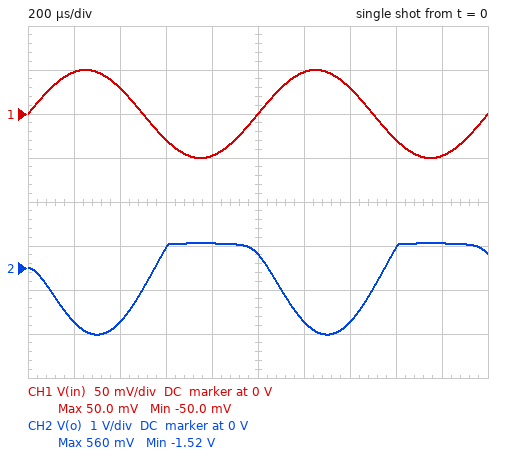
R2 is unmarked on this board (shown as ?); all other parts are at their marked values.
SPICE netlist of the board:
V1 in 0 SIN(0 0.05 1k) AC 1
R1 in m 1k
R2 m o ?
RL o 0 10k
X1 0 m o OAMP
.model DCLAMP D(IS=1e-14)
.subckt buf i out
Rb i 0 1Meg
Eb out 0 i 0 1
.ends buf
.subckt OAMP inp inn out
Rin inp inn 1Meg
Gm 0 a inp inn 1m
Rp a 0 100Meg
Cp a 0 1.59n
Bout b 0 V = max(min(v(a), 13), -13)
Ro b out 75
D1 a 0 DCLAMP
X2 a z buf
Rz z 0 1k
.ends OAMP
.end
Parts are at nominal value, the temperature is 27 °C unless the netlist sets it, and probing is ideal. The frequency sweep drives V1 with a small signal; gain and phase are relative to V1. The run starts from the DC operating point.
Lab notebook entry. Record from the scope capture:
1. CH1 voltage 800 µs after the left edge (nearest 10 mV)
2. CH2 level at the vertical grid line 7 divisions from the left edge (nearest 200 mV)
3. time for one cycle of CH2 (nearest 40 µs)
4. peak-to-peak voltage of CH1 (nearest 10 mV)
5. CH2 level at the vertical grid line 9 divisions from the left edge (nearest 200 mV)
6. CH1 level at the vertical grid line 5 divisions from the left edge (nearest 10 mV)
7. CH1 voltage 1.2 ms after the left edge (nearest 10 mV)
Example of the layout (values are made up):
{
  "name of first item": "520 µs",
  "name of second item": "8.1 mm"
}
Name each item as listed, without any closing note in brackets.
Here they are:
{
  "CH1 voltage 800 µs after the left edge": "-50 mV",
  "CH2 level at the vertical grid line 7 divisions from the left edge": "-1.2 V",
  "time for one cycle of CH2": "1.00 ms",
  "peak-to-peak voltage of CH1": "100 mV",
  "CH2 level at the vertical grid line 9 divisions from the left edge": "600 mV",
  "CH1 level at the vertical grid line 5 divisions from the left edge": "0 V",
  "CH1 voltage 1.2 ms after the left edge": "50 mV"
}
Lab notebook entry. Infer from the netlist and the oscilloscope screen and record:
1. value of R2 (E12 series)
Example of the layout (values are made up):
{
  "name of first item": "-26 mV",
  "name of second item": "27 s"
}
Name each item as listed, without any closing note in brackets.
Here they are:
{
  "value of R2": "33 kΩ"
}
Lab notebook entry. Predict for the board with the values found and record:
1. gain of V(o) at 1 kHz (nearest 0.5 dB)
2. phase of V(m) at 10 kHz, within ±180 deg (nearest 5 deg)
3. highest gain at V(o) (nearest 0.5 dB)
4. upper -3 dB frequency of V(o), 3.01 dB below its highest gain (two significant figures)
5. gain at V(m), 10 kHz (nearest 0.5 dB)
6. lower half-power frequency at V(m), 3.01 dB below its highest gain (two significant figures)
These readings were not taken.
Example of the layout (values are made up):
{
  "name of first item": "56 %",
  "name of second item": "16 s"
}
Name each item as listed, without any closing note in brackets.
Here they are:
{
  "gain of V(o) at 1 kHz": "29.5 dB",
  "phase of V(m) at 10 kHz, within ±180 deg": "15 deg",
  "highest gain at V(o)": "30.0 dB",
  "upper -3 dB frequency of V(o), 3.01 dB below its highest gain": "3.0 kHz",
  "gain at V(m), 10 kHz": "-0.5 dB",
  "lower half-power frequency at V(m), 3.01 dB below its highest gain": "3.0 kHz"
}
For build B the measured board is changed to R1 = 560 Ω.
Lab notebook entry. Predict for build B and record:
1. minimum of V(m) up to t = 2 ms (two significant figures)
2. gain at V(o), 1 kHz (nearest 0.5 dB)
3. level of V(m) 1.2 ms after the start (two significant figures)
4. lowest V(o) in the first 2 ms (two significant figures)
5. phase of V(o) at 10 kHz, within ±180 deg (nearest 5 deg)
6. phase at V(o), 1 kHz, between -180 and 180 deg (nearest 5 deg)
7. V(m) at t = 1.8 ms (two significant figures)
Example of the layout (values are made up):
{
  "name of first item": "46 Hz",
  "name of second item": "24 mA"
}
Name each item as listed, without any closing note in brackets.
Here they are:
{
  "minimum of V(m) up to t = 2 ms": "-40 mV",
  "gain at V(o), 1 kHz": "33.5 dB",
  "level of V(m) 1.2 ms after the start": "18 mV",
  "lowest V(o) in the first 2 ms": "-2.4 V",
  "phase of V(o) at 10 kHz, within ±180 deg": "100 deg",
  "phase at V(o), 1 kHz, between -180 and 180 deg": "150 deg",
  "V(m) at t = 1.8 ms": "-37 mV"
}
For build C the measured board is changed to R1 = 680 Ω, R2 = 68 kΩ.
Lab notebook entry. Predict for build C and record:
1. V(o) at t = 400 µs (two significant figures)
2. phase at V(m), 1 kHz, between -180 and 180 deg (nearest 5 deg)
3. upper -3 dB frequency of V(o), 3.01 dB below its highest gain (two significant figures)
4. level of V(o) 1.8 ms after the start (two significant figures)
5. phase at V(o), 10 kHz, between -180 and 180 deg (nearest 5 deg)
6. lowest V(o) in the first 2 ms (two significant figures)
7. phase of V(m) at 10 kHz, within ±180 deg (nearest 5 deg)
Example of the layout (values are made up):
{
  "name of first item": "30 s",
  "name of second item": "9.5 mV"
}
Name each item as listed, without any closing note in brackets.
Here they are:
{
  "V(o) at t = 400 µs": "-3.4 V",
  "phase at V(m), 1 kHz, between -180 and 180 deg": "40 deg",
  "upper -3 dB frequency of V(o), 3.01 dB below its highest gain": "1.1 kHz",
  "level of V(o) 1.8 ms after the start": "570 mV",
  "phase at V(o), 10 kHz, between -180 and 180 deg": "95 deg",
  "lowest V(o) in the first 2 ms": "-3.5 V",
  "phase of V(m) at 10 kHz, within ±180 deg": "5 deg"
}
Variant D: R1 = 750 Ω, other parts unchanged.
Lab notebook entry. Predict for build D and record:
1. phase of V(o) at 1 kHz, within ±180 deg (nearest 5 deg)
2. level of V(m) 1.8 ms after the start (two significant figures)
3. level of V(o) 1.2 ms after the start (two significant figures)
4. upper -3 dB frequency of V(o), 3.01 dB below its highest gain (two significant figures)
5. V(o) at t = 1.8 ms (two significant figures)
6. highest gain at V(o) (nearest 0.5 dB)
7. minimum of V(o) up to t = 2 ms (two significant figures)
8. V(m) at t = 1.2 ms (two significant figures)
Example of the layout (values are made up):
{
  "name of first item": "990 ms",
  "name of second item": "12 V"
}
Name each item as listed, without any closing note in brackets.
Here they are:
{
  "phase of V(o) at 1 kHz, within ±180 deg": "155 deg",
  "level of V(m) 1.8 ms after the start": "-34 mV",
  "level of V(o) 1.2 ms after the start": "-1.5 V",
  "upper -3 dB frequency of V(o), 3.01 dB below its highest gain": "2.3 kHz",
  "V(o) at t = 1.8 ms": "560 mV",
  "highest gain at V(o)": "32.5 dB",
  "minimum of V(o) up to t = 2 ms": "-1.9 V",
  "V(m) at t = 1.2 ms": "14 mV"
}
